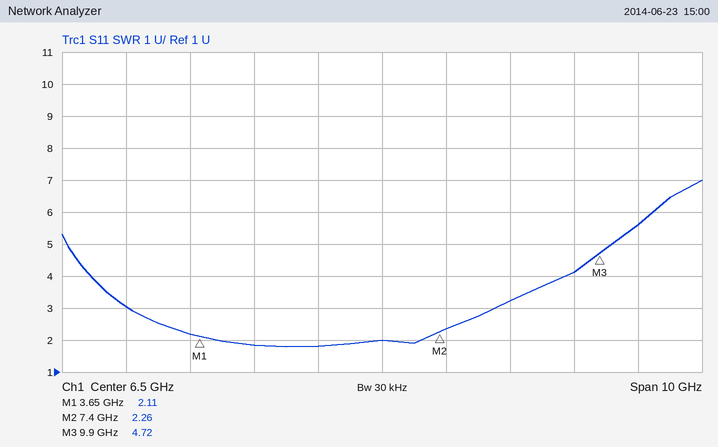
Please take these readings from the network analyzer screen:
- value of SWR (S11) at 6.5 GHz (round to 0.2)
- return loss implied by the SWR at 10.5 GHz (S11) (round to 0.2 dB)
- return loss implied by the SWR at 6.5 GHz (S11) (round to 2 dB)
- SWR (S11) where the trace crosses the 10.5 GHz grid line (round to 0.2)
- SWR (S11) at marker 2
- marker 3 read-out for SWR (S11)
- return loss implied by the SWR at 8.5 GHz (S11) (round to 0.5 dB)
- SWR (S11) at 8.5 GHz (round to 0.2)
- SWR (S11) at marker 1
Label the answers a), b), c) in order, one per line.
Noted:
a) 2.0
b) 3.2 dB
c) 10 dB
d) 5.6
e) 2.26
f) 4.72
g) 5.5 dB
h) 3.2
i) 2.11
